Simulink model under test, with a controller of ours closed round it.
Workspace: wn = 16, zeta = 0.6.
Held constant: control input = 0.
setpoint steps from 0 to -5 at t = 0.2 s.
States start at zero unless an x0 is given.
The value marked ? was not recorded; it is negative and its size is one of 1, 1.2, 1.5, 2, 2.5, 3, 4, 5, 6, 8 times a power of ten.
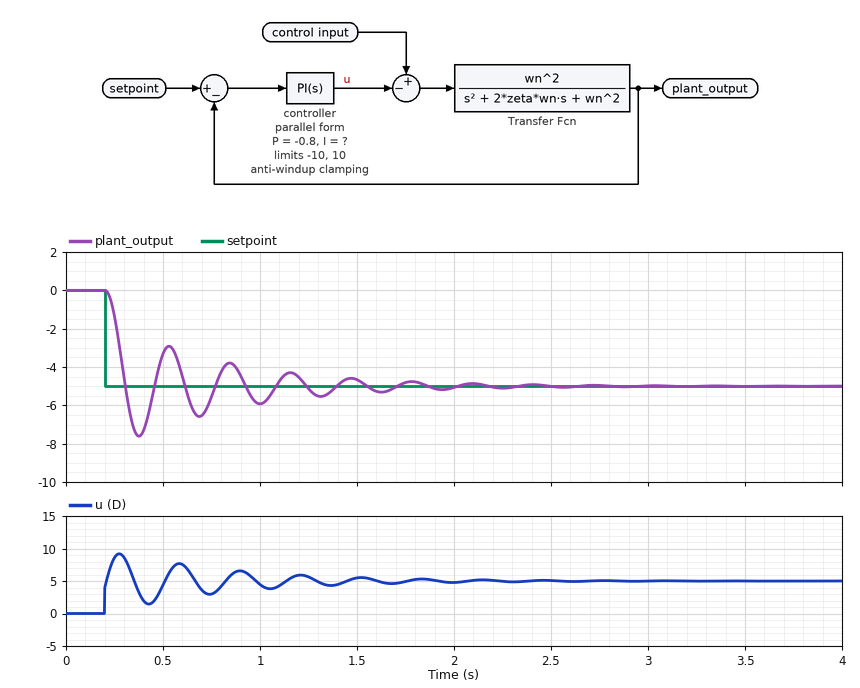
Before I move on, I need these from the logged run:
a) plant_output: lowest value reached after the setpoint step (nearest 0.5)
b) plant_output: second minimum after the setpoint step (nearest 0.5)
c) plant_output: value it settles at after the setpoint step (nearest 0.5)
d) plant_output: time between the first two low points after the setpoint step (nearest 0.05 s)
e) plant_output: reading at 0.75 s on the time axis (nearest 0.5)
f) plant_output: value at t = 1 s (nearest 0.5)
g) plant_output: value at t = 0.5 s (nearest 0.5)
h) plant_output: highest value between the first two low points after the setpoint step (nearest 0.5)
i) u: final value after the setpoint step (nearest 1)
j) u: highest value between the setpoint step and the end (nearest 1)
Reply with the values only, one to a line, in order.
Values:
-7.5
-6.5
-5.0
0.30 s
-5.5
-6.0
-3.5
-3.0
5
9
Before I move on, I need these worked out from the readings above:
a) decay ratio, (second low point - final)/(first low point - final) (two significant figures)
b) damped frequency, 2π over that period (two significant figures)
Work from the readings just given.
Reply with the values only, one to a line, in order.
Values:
0.60
21 rad/s
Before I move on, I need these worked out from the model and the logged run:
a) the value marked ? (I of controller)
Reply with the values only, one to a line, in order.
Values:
-25
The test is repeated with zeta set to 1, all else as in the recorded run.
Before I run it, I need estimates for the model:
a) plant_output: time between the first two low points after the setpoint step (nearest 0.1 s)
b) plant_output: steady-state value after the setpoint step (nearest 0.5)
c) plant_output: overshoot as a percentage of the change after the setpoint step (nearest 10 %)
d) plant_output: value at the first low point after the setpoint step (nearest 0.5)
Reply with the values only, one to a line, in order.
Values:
0.4 s
-5.0
40 %
-7.0
